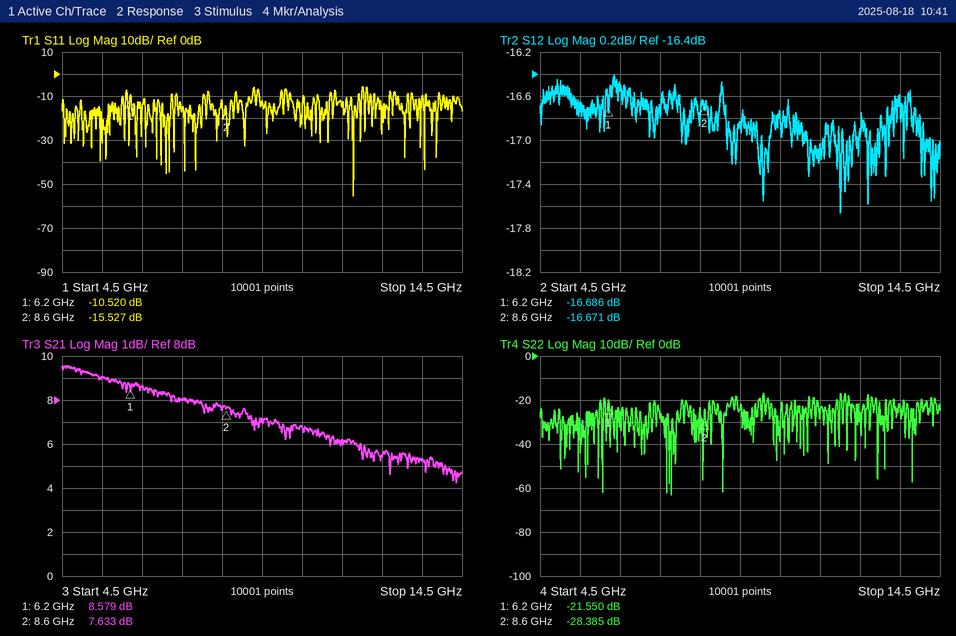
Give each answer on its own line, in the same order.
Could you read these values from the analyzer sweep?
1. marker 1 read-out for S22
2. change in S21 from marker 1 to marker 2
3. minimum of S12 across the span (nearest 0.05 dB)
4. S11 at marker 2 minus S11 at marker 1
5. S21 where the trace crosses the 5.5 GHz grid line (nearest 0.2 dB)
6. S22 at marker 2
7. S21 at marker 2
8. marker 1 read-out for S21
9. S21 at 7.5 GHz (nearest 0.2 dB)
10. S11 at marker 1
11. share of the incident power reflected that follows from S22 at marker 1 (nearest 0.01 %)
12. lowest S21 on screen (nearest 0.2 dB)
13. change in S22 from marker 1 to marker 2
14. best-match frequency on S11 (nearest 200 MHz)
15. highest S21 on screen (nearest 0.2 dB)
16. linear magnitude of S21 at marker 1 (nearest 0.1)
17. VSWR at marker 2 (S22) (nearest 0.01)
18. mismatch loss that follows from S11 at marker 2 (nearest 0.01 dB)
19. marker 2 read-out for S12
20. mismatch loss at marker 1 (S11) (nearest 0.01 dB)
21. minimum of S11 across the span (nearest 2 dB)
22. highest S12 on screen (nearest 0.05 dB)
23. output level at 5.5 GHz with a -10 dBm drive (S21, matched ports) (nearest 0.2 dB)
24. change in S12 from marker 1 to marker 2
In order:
-21.550 dB
-0.946 dB
-17.65 dB
-5.007 dB
9.0 dB
-28.385 dB
7.633 dB
8.579 dB
8.0 dB
-10.520 dB
0.70 %
4.2 dB
-6.835 dB
11.8 GHz
9.6 dB
2.7
1.08
0.12 dB
-16.671 dB
0.40 dB
-56 dB
-16.40 dB
-1.0 dBm
0.015 dB
